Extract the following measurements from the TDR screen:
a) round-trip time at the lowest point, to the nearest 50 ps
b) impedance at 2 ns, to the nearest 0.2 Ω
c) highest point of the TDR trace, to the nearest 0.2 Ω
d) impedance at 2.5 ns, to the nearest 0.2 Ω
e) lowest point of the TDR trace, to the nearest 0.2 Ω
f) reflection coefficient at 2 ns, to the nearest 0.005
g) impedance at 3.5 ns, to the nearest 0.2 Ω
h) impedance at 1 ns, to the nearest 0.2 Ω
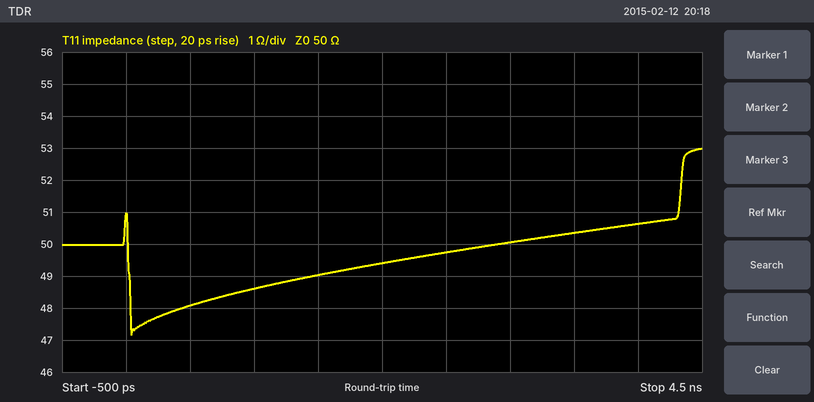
50 ps
49.4 Ω
53.0 Ω
49.8 Ω
47.2 Ω
-0.005
50.4 Ω
48.6 Ω
